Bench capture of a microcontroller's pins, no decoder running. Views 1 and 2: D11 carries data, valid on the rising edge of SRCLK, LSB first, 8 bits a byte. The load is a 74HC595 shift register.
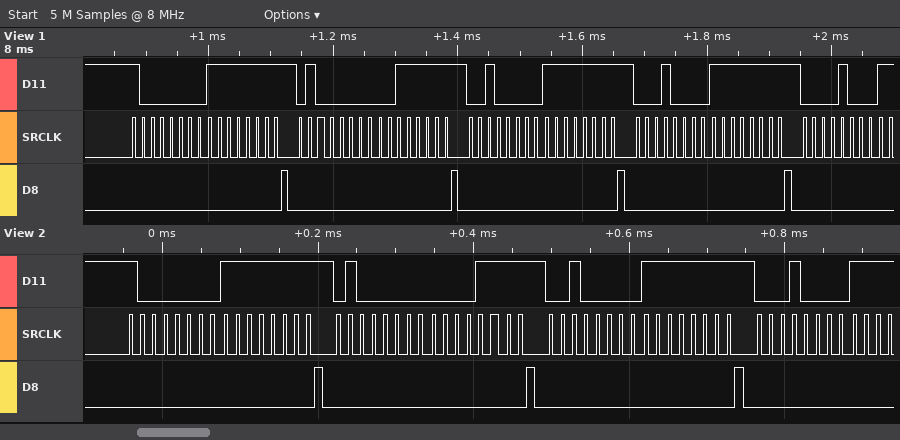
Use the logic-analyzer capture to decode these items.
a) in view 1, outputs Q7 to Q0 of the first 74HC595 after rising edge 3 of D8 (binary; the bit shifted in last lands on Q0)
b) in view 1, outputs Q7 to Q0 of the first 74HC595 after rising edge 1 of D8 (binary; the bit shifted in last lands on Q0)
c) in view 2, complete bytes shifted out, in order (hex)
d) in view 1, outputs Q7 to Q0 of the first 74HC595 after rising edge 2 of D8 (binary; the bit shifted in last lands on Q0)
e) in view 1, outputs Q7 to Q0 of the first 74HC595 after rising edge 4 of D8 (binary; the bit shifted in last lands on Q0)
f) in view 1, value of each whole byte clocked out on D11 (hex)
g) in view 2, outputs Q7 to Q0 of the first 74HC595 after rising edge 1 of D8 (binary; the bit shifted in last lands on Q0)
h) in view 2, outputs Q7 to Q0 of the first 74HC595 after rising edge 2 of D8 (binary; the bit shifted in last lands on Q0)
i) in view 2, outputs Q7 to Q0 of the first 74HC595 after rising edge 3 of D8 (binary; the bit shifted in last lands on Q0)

11111111
11111111
01 FF 02 F0 04 FF 08
00111111
11111111
0x01 0xFF 0x02 0xFC 0x04 0xFF 0x08 0xFF 0x10
11111111
00001111
11111111
